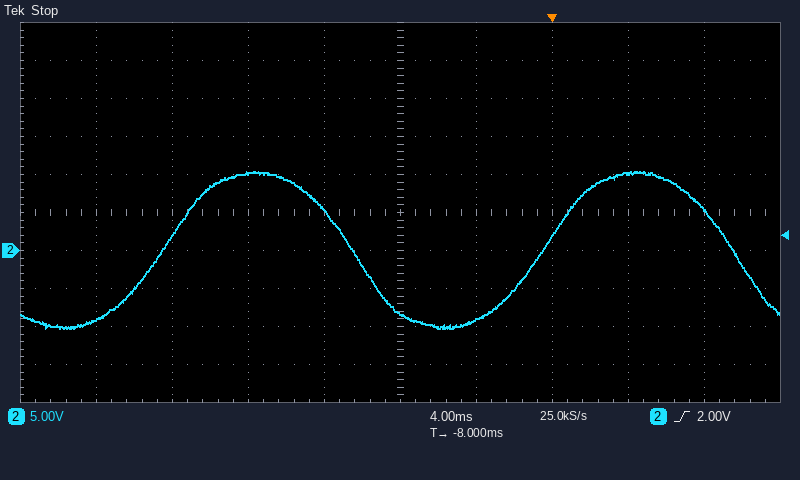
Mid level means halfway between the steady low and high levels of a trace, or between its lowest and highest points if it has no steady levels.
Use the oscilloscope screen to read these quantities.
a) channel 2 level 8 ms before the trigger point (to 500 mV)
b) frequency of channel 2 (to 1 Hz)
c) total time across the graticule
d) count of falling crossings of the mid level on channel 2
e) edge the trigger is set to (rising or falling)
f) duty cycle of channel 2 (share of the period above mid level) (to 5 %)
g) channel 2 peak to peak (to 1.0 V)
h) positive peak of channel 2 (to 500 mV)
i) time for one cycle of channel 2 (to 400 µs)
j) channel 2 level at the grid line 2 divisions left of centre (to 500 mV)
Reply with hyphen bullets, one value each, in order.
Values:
- -8.5 V
- 50 Hz
- 40 ms
- 2
- rising
- 50 %
- 21.0 V
- 10.5 V
- 20.0 ms
- 10.0 V
